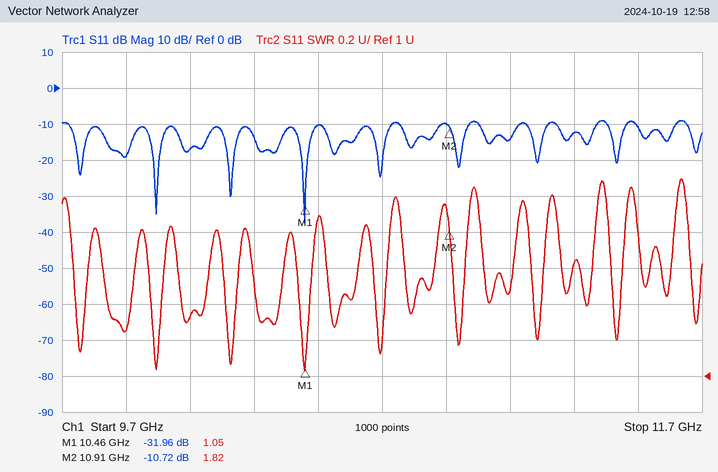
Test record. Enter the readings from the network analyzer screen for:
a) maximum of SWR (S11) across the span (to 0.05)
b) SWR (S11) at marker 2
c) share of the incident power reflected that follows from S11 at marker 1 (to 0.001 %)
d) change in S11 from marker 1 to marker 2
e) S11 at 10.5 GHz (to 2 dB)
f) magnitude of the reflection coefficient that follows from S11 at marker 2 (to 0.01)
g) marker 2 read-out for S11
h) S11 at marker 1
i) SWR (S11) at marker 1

2.10
1.82
0.064 %
21.24 dB
-10 dB
0.29
-10.72 dB
-31.96 dB
1.05
